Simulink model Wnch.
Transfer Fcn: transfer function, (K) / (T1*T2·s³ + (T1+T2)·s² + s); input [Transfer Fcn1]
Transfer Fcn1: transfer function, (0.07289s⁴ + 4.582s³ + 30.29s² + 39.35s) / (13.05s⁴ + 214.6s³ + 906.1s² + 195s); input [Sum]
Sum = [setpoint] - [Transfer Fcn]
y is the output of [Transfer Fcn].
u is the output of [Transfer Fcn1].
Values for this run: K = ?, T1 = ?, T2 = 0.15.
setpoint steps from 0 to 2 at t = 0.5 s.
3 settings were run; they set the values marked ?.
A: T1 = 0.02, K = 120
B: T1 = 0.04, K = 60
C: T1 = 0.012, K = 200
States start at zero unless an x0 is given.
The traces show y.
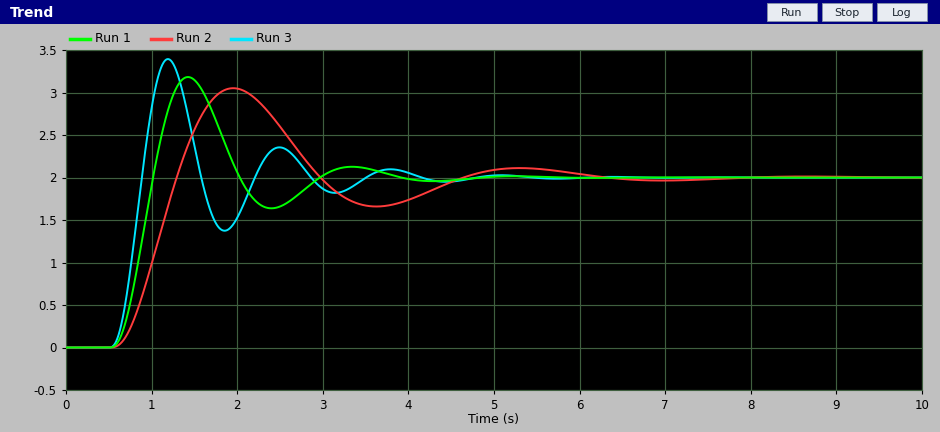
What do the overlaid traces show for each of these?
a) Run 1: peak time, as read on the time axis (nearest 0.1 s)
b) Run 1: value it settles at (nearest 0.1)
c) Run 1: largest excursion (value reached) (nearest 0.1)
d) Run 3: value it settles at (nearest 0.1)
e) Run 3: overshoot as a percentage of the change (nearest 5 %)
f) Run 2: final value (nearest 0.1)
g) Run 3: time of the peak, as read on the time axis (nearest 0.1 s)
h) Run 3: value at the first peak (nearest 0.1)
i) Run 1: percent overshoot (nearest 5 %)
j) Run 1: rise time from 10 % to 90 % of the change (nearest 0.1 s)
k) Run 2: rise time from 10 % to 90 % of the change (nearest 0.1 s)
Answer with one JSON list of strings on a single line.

["1.4 s", "2.0", "3.2", "2.0", "70 %", "2.0", "1.2 s", "3.4", "60 %", "0.3 s", "0.5 s"]
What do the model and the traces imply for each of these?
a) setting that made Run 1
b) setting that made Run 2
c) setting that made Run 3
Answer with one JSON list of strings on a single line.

["A", "B", "C"]
